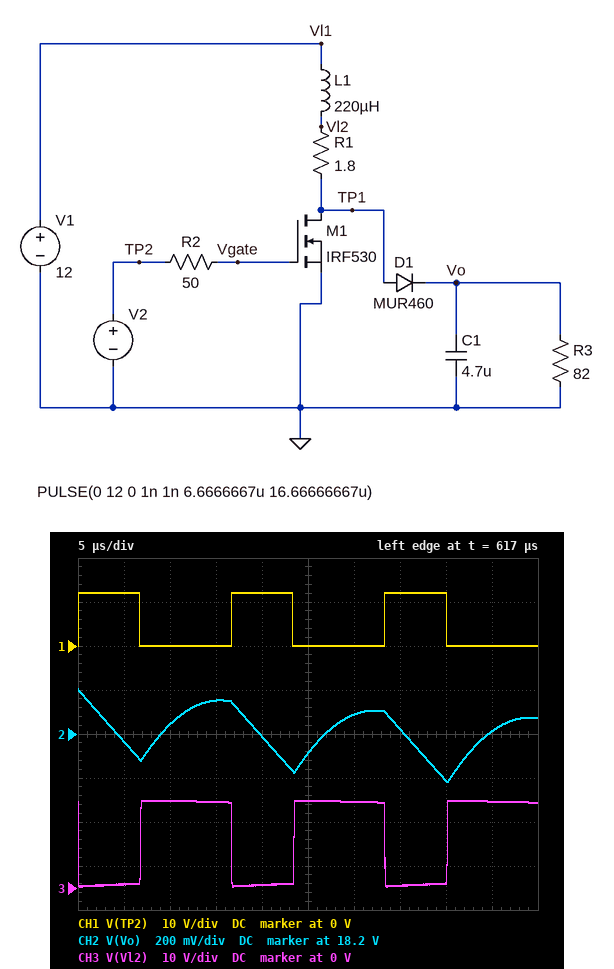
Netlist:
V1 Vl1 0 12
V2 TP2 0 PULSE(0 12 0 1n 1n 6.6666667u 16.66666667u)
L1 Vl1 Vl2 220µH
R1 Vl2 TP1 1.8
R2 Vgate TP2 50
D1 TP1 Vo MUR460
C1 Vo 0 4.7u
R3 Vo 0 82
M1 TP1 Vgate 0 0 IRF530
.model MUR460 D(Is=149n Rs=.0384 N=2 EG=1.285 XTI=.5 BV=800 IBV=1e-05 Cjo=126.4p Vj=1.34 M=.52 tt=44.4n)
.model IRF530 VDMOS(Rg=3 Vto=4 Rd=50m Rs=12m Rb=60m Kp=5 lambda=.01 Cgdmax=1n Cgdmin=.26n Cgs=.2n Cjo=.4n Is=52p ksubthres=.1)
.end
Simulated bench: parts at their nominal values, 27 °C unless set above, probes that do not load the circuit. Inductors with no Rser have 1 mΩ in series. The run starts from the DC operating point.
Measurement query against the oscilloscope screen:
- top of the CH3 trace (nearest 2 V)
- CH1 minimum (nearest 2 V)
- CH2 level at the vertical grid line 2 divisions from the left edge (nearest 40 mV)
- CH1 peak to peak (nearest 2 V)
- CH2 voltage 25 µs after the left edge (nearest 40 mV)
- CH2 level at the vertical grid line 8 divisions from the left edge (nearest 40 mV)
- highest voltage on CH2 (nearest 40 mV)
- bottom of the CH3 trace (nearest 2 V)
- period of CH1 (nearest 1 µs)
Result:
20 V
0 V
18.24 V
12 V
18.12 V
18.00 V
18.40 V
0 V
17 µs
